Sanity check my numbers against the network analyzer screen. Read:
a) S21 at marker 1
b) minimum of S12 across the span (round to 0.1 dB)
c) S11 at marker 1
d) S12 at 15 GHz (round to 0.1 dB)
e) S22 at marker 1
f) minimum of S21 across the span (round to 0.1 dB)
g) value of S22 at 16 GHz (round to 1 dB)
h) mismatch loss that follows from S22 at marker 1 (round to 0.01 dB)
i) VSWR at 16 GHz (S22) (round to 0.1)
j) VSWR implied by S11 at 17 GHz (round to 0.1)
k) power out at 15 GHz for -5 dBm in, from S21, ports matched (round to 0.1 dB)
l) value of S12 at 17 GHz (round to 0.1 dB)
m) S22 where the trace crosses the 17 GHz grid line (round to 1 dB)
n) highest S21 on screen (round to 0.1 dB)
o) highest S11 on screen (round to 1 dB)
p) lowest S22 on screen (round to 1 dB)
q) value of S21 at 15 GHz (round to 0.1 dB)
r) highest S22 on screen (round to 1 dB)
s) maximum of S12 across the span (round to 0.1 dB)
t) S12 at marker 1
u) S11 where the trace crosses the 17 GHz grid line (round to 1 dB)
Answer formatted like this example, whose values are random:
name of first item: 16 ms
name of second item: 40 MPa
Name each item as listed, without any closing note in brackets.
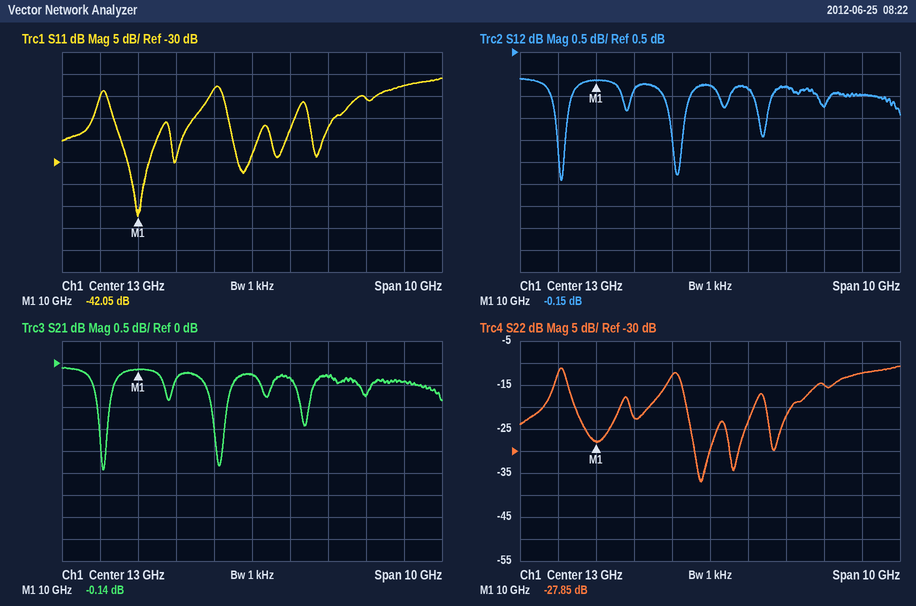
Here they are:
S21 at marker 1: -0.14 dB
minimum of S12 across the span: -2.4 dB
S11 at marker 1: -42.05 dB
S12 at 15 GHz: -0.3 dB
S22 at marker 1: -27.85 dB
minimum of S21 across the span: -2.4 dB
value of S22 at 16 GHz: -15 dB
mismatch loss that follows from S22 at marker 1: 0.01 dB
VSWR at 16 GHz (S22): 1.4
VSWR implied by S11 at 17 GHz: 1.6
power out at 15 GHz for -5 dBm in, from S21, ports matched: -5.3 dBm
value of S12 at 17 GHz: -0.5 dB
S22 where the trace crosses the 17 GHz grid line: -12 dB
highest S21 on screen: -0.1 dB
highest S11 on screen: -11 dB
lowest S22 on screen: -37 dB
value of S21 at 15 GHz: -0.3 dB
highest S22 on screen: -11 dB
maximum of S12 across the span: -0.1 dB
S12 at marker 1: -0.15 dB
S11 where the trace crosses the 17 GHz grid line: -13 dB
